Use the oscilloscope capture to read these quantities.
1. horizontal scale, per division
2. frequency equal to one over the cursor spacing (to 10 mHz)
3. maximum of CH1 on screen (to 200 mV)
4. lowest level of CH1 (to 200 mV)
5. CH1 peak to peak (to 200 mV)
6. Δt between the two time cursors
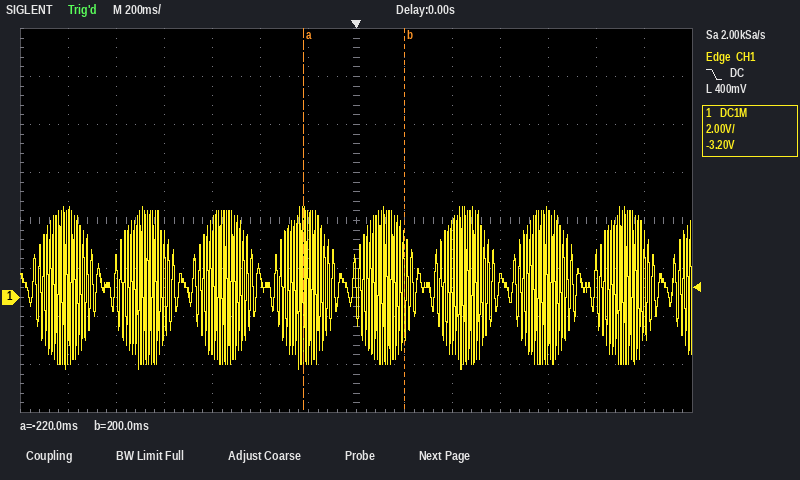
200 ms
2.38 Hz
3.8 V
-3.0 V
6.8 V
420 ms
